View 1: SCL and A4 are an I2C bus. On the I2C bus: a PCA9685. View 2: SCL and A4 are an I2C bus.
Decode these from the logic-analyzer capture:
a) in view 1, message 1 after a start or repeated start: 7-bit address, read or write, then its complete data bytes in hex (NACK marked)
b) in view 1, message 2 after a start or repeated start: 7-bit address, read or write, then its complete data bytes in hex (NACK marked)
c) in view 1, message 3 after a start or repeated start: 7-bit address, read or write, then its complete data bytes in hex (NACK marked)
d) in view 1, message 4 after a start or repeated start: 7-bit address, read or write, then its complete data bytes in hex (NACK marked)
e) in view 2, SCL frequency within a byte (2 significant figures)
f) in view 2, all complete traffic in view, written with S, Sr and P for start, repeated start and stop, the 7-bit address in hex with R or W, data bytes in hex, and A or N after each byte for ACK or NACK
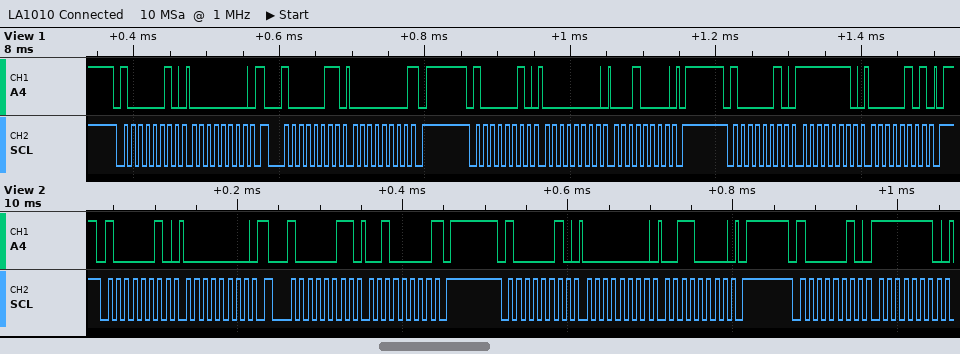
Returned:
0x41 write: 00
0x41 read: 00 NACK
0x41 write: 00 10
0x41 write: FE 05
100 kHz
S 41W A 00 A Sr 41R A 20 N P S 41W A 00 A 30 A P S 41W A FE A
